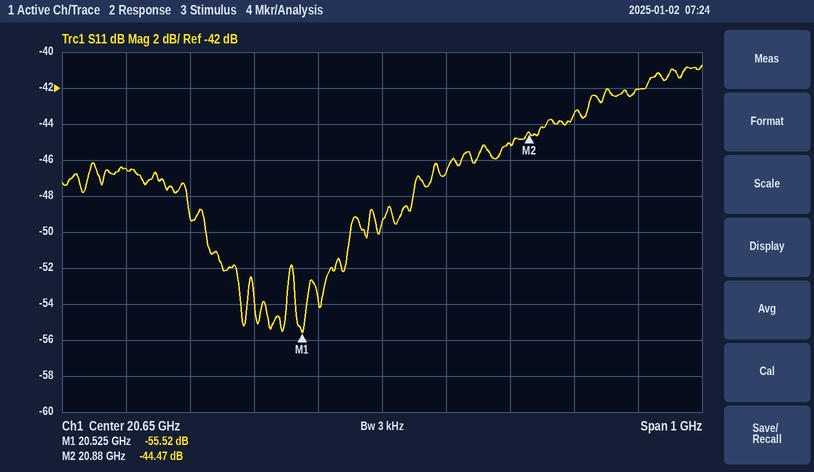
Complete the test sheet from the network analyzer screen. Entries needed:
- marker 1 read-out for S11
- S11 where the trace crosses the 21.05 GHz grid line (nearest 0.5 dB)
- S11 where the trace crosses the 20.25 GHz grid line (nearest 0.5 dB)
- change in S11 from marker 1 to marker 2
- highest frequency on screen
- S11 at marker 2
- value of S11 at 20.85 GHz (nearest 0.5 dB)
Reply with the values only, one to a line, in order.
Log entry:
-55.52 dB
-42.0 dB
-46.5 dB
11.05 dB
21.15 GHz
-44.47 dB
-45.0 dB
